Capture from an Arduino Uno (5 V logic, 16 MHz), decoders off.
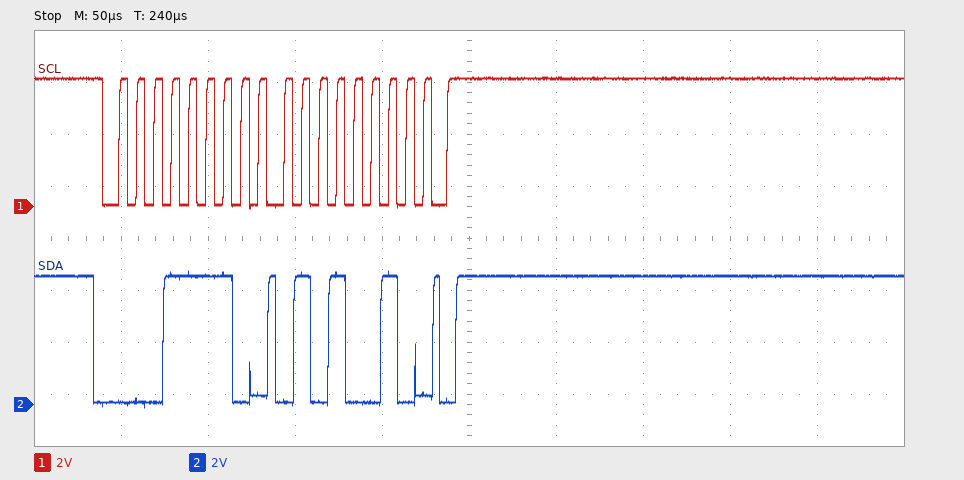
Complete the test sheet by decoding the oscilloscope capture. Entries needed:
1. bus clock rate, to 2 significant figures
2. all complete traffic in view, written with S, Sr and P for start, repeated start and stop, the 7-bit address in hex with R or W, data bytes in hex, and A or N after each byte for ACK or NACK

100 kHz
S 0FW A 52 A P
